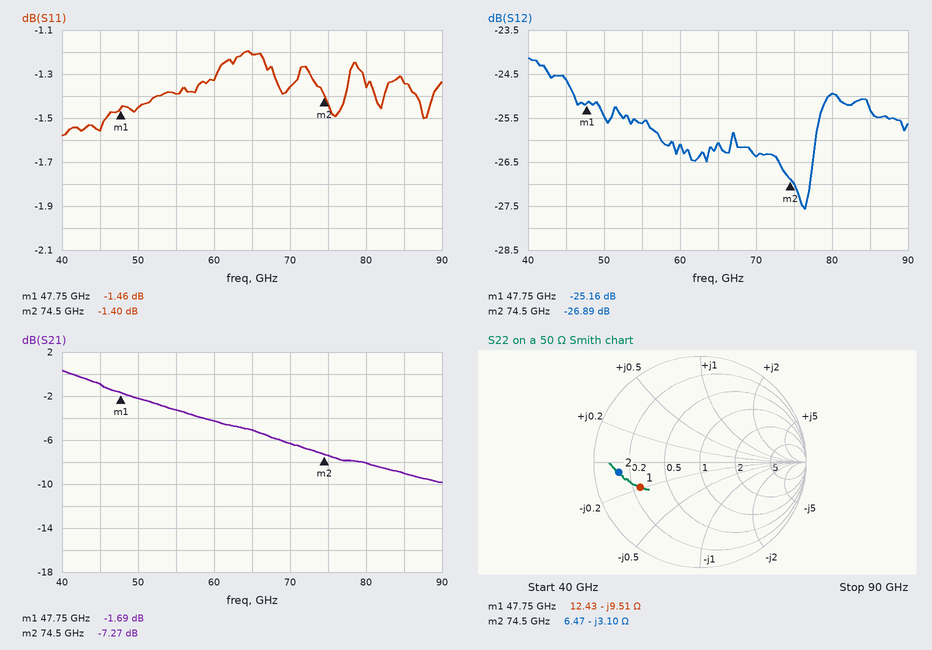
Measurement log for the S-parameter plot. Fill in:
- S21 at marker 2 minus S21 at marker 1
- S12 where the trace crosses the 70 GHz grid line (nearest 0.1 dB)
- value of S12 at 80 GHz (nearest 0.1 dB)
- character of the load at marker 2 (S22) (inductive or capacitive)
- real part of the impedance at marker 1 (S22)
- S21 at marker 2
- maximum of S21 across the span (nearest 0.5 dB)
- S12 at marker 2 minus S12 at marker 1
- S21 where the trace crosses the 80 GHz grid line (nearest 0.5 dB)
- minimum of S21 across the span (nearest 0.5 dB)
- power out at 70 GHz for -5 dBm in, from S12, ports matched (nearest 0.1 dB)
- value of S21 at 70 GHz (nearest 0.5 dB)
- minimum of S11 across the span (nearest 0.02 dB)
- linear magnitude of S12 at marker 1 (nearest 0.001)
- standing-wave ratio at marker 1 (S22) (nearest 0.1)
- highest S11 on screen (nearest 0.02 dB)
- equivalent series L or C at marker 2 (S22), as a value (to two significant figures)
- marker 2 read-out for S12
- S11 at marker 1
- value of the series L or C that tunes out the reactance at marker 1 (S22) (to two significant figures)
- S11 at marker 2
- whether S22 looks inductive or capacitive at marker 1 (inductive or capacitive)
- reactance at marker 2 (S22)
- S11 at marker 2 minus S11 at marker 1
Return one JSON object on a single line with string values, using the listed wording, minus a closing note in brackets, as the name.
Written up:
{"S21 at marker 2 minus S21 at marker 1": "-5.58 dB", "S12 where the trace crosses the 70 GHz grid line": "-26.4 dB", "value of S12 at 80 GHz": "-24.9 dB", "character of the load at marker 2 (S22)": "capacitive", "real part of the impedance at marker 1": "12.43 Ω", "S21 at marker 2": "-7.27 dB", "maximum of S21 across the span": "0.5 dB", "S12 at marker 2 minus S12 at marker 1": "-1.73 dB", "S21 where the trace crosses the 80 GHz grid line": "-8.0 dB", "minimum of S21 across the span": "-10.0 dB", "power out at 70 GHz for -5 dBm in, from S12, ports matched": "-31.4 dBm", "value of S21 at 70 GHz": "-6.5 dB", "minimum of S11 across the span": "-1.58 dB", "linear magnitude of S12 at marker 1": "0.055", "standing-wave ratio at marker 1 (S22)": "4.2", "highest S11 on screen": "-1.20 dB", "equivalent series L or C at marker 2 (S22), as a value": "690 fF", "marker 2 read-out for S12": "-26.89 dB", "S11 at marker 1": "-1.46 dB", "value of the series L or C that tunes out the reactance at marker 1 (S22)": "32 pH", "S11 at marker 2": "-1.40 dB", "whether S22 looks inductive or capacitive at marker 1": "capacitive", "reactance at marker 2": "-3.10 Ω", "S11 at marker 2 minus S11 at marker 1": "0.06 dB"}
